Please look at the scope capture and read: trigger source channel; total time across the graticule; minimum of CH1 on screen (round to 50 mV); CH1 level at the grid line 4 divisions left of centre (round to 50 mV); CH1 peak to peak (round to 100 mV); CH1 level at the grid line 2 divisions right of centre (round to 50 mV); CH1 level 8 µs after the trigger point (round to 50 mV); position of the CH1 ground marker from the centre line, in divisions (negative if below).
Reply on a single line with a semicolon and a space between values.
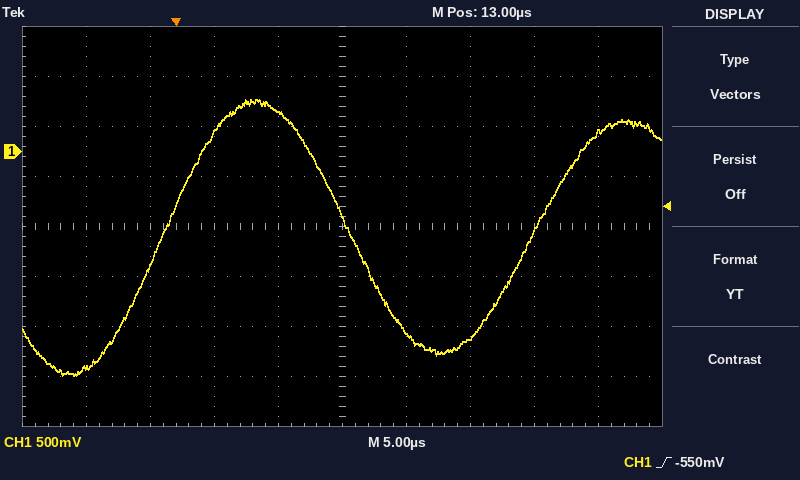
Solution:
CH1; 50 µs; -2.25 V; -2.15 V; 2.80 V; -1.85 V; 400 mV; +1.5 div
